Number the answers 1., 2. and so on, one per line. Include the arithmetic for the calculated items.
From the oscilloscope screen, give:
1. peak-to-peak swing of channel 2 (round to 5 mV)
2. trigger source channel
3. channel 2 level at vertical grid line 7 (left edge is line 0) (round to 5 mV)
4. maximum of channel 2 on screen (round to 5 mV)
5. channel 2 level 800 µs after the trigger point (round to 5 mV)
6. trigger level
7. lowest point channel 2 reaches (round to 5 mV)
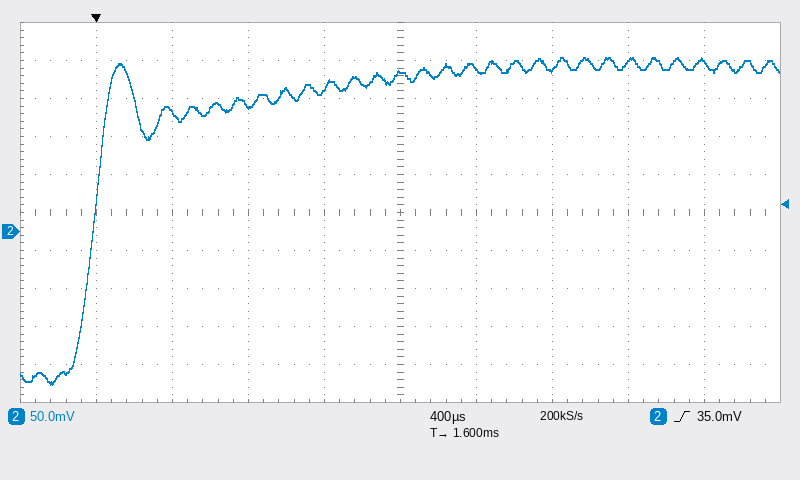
1. 230 mV − (-200 mV) = 430 mV
2. channel 2
3. 215 mV
4. 230 mV
5. 165 mV
6. 35.0 mV
7. -200 mV
